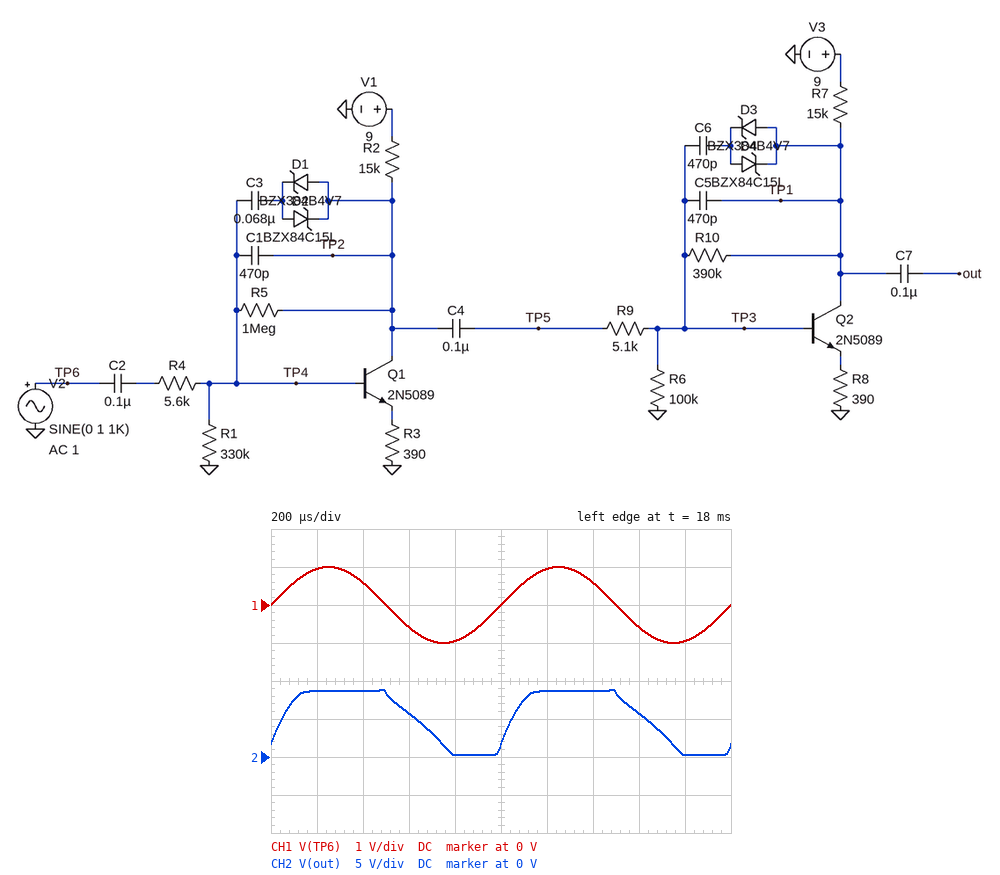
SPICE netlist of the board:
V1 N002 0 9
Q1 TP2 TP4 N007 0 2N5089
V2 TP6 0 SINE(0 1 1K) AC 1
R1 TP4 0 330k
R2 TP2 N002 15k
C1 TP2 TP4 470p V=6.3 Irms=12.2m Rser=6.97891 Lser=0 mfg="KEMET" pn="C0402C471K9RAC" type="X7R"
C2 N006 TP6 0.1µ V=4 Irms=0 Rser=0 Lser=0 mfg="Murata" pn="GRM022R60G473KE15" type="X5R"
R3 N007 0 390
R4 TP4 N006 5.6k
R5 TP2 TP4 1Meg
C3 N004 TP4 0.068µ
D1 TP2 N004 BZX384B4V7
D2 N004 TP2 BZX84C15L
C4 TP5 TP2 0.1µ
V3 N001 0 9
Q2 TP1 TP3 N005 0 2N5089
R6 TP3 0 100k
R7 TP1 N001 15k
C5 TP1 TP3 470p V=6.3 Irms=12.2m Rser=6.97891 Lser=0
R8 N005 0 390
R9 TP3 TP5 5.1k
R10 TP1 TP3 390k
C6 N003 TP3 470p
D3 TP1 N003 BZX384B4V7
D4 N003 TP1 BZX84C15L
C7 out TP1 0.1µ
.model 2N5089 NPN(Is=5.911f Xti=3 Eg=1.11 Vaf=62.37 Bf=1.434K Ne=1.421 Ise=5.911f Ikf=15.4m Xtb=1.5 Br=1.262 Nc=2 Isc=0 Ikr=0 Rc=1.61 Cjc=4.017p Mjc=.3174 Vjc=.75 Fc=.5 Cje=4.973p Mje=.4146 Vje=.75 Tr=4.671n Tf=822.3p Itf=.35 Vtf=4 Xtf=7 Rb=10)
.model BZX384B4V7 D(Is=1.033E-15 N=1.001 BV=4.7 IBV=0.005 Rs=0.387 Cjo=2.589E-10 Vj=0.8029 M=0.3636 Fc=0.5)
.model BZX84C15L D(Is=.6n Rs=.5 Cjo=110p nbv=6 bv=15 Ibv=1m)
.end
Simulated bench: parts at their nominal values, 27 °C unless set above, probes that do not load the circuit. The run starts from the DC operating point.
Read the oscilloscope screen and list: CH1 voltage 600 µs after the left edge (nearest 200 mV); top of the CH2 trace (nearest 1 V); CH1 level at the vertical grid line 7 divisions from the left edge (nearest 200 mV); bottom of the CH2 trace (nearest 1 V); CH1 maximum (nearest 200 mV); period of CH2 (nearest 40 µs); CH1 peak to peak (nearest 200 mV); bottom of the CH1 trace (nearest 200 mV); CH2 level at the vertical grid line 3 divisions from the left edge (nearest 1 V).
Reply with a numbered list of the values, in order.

1. -600 mV
2. 9 V
3. 600 mV
4. 0 V
5. 1.0 V
6. 1.00 ms
7. 2.0 V
8. -1.0 V
9. 6 V
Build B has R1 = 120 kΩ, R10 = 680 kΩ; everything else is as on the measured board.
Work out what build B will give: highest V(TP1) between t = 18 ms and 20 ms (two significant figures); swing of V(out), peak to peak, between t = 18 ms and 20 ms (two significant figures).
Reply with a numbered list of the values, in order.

1. 9.0 V
2. 8.7 V
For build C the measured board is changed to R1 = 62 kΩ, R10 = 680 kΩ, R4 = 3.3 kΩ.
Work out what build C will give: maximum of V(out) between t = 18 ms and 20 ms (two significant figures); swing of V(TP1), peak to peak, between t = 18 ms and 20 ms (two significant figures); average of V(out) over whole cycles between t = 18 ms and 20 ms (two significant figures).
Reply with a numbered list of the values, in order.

1. 9.1 V
2. 8.8 V
3. 5.5 V
